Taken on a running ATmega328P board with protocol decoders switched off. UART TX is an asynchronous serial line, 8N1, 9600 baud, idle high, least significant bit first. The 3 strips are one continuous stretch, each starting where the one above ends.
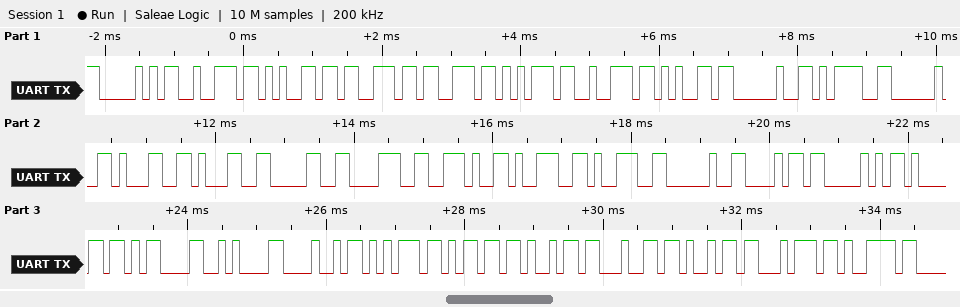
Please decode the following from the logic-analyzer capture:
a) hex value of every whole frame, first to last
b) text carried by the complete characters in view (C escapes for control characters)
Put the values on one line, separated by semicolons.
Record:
50 72 65 73 73 75 72 65 20 3D 20 31 31 30 38 2E 39 39 20 68 50 61 0D 0A 48 75 6D 69 64 69 74 79; "Pressure = 1108.99 hPa\r\nHumidity"
